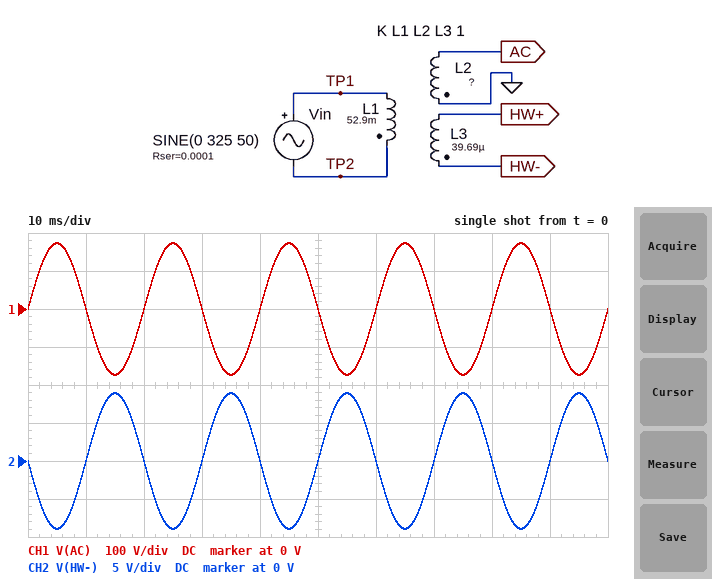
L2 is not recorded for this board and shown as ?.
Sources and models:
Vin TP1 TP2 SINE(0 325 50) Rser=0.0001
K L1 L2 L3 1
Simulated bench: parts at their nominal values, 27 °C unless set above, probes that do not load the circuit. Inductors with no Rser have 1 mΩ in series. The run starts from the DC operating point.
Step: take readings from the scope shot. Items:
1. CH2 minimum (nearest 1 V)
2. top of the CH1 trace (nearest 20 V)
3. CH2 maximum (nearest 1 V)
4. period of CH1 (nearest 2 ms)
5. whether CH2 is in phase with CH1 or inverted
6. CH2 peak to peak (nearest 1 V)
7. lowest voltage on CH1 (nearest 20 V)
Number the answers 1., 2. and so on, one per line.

1. -9 V
2. 180 V
3. 9 V
4. 20 ms
5. inverted
6. 18 V
7. -180 V
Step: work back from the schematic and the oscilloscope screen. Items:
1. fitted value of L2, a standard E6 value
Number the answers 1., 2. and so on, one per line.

1. 15 mH
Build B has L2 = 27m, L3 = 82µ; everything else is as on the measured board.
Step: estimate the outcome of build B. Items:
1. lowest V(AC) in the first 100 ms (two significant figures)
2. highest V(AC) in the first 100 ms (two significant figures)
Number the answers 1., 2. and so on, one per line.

1. -230 V
2. 230 V
